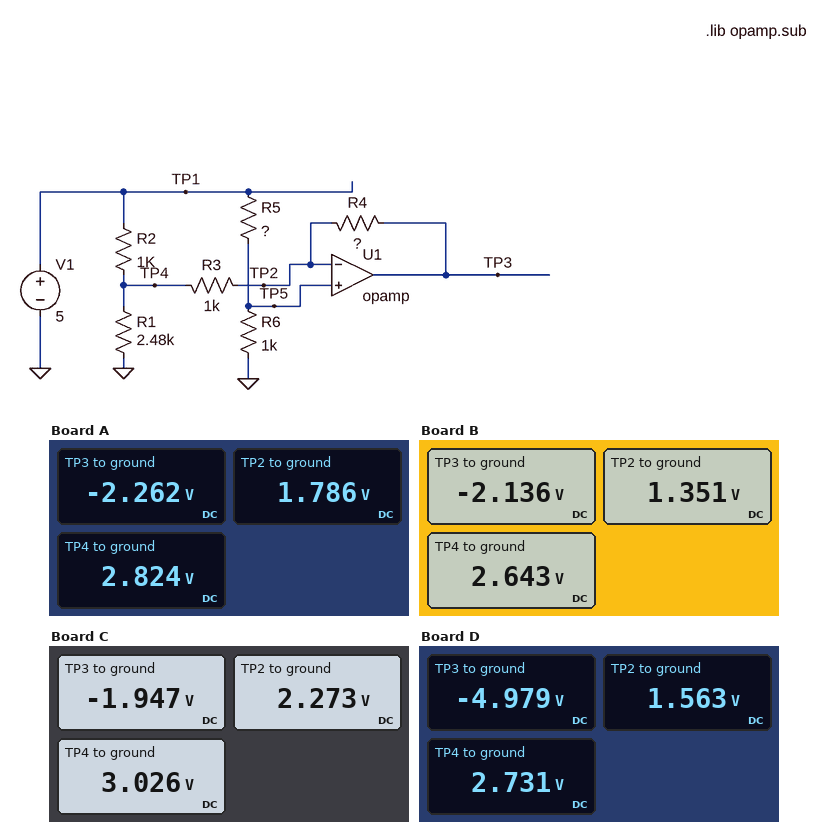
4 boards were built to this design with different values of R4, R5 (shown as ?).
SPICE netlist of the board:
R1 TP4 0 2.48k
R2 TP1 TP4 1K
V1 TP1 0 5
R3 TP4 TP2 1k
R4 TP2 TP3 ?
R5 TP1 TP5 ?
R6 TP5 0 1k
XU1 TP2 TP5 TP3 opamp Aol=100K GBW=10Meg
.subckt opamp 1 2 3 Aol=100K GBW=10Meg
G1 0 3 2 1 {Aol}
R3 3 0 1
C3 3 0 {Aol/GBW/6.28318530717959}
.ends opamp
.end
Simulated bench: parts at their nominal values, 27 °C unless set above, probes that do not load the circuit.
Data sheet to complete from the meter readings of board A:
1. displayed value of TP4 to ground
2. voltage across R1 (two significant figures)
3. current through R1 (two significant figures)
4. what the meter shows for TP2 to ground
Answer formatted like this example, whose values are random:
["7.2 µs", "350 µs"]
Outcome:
["2.824 V", "2.8 V", "1.1 mA", "1.786 V"]
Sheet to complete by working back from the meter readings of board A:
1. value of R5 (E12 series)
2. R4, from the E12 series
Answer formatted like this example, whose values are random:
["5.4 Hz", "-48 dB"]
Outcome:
["1.8 kΩ", "3.9 kΩ"]
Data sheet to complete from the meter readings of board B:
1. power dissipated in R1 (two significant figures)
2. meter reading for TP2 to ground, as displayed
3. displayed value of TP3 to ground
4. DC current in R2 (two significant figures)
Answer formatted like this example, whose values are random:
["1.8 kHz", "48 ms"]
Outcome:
["2.8 mW", "1.351 V", "-2.136 V", "2.4 mA"]
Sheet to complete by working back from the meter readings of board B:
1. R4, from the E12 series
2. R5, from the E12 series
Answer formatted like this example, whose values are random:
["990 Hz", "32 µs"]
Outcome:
["2.7 kΩ", "2.7 kΩ"]
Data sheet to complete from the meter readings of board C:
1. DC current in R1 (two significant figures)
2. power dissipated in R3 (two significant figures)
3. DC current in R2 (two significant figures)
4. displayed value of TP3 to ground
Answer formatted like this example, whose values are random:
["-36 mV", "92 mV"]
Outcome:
["1.2 mA", "570 µW", "2.0 mA", "-1.947 V"]
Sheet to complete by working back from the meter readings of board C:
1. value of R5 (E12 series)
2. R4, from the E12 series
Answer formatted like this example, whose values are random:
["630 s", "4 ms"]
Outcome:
["1.2 kΩ", "5.6 kΩ"]
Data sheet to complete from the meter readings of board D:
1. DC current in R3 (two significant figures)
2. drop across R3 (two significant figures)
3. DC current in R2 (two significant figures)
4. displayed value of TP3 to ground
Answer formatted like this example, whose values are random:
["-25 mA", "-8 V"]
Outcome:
["1.2 mA", "1.2 V", "2.3 mA", "-4.979 V"]
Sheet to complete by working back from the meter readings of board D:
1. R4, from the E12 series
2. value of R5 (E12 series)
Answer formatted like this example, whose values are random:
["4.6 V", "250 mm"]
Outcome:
["5.6 kΩ", "2.2 kΩ"]
